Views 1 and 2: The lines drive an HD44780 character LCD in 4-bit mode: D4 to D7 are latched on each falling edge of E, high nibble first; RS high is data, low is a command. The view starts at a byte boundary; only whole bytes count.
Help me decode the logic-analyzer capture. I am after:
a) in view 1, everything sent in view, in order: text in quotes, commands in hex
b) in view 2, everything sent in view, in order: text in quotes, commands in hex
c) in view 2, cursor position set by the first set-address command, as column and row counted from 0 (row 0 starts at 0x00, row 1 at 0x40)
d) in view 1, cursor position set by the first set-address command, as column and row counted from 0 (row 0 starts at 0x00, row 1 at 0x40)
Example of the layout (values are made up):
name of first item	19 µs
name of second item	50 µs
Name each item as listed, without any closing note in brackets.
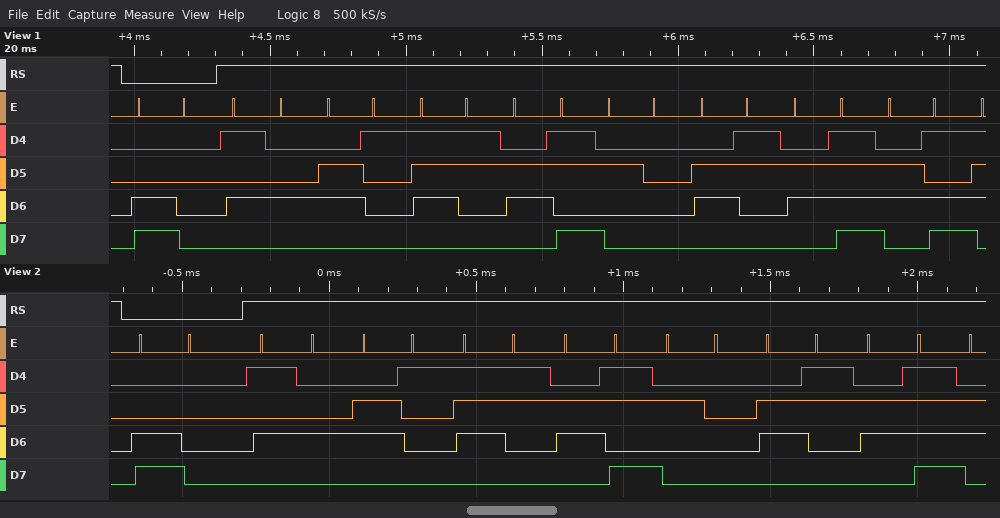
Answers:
in view 1, everything sent in view, in order: text in quotes, commands in hex	0xC0 "Task com"
in view 2, everything sent in view, in order: text in quotes, commands in hex	0xC0 "Task co"
in view 2, cursor position set by the first set-address command, as column and row counted from 0	column 0, row 1
in view 1, cursor position set by the first set-address command, as column and row counted from 0	column 0, row 1
